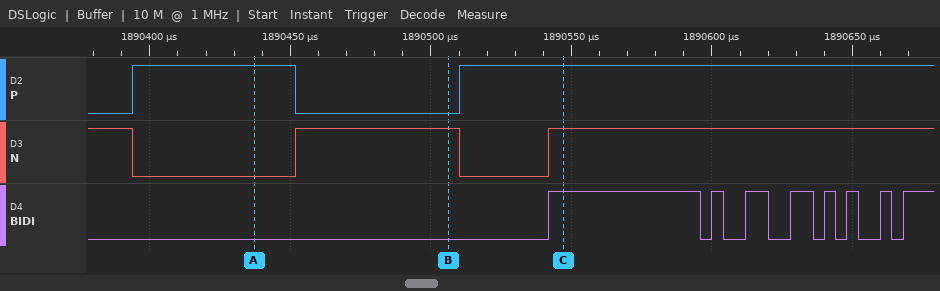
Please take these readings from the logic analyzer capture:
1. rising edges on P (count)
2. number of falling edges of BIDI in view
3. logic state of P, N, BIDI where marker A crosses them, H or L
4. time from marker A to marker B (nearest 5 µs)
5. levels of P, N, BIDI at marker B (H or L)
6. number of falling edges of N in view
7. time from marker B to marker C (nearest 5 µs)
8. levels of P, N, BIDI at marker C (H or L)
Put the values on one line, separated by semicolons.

2; 7; P=H, N=L, BIDI=L; 70 µs; P=L, N=H, BIDI=L; 2; 40 µs; P=H, N=H, BIDI=H
